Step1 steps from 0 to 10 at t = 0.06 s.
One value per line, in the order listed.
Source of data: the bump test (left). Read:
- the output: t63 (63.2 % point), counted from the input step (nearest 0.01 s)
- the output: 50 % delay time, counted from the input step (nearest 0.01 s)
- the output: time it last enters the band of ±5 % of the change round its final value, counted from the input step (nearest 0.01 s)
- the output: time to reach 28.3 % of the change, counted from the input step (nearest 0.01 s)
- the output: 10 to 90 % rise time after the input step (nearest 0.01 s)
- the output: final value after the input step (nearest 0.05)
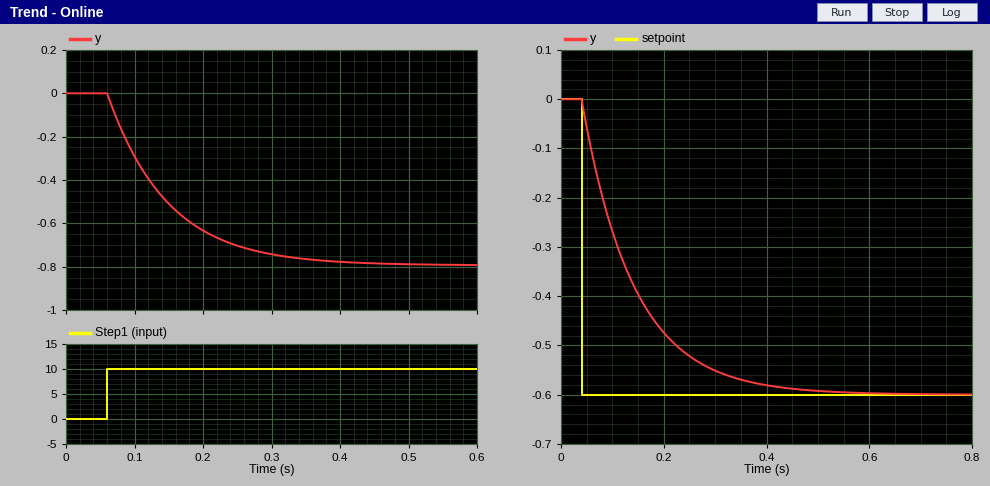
0.09 s
0.06 s
0.26 s
0.03 s
0.19 s
-0.80
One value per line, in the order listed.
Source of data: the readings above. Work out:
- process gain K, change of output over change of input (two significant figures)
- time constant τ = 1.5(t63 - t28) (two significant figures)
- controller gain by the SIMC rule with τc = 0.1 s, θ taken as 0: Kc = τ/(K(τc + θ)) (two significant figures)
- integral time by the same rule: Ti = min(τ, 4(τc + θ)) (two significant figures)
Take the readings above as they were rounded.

-0.080
0.090 s
-11
0.090 s
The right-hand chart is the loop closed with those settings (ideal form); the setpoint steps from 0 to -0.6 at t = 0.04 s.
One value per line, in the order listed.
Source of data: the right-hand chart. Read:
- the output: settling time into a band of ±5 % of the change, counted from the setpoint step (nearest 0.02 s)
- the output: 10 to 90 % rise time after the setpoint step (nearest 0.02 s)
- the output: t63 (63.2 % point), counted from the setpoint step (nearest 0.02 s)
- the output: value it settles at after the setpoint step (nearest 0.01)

0.32 s
0.22 s
0.10 s
-0.60
